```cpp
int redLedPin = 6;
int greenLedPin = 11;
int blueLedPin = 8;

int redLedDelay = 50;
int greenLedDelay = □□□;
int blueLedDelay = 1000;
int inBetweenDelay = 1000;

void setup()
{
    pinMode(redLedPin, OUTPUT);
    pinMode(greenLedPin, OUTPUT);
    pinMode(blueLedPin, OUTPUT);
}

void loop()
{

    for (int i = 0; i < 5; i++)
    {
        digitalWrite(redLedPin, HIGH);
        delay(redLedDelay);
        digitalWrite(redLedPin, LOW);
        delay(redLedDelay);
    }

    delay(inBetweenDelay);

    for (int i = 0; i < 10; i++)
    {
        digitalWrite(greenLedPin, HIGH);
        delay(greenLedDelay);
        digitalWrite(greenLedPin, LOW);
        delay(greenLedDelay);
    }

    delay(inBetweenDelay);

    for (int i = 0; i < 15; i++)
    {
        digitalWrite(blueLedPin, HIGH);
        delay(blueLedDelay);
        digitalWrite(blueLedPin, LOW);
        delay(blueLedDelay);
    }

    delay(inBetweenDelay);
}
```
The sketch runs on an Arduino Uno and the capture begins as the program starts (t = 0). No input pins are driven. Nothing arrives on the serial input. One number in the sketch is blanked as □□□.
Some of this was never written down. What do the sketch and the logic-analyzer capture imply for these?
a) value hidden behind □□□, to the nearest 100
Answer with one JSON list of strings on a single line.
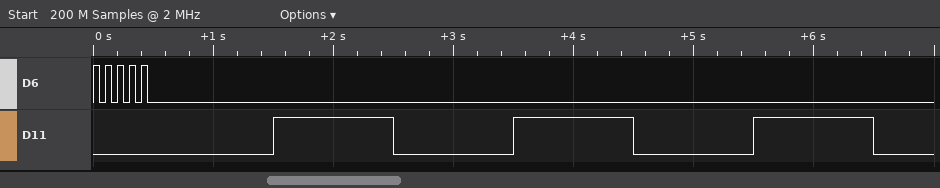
["1000"]
